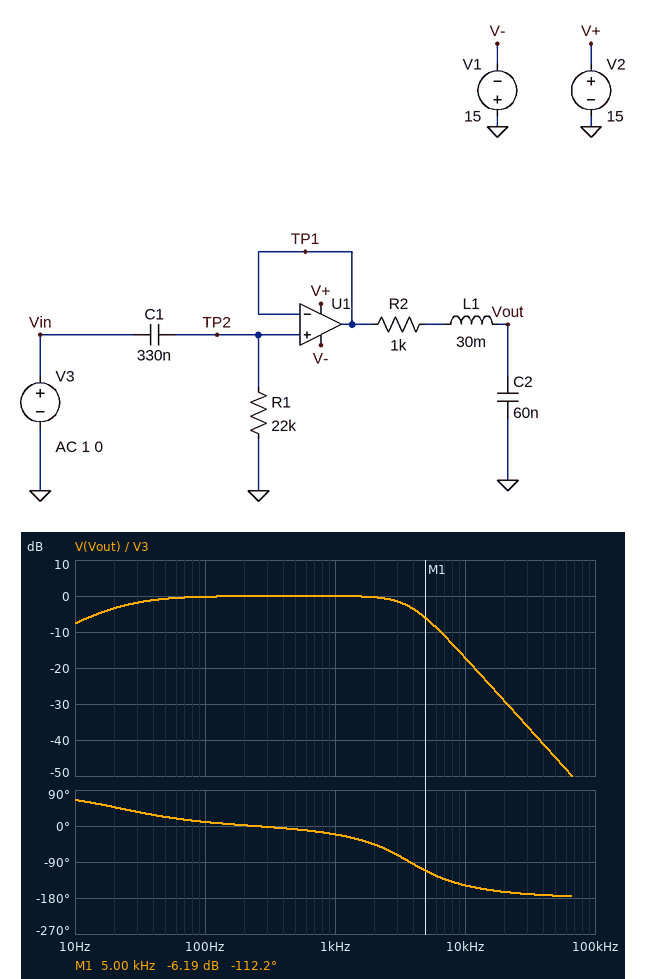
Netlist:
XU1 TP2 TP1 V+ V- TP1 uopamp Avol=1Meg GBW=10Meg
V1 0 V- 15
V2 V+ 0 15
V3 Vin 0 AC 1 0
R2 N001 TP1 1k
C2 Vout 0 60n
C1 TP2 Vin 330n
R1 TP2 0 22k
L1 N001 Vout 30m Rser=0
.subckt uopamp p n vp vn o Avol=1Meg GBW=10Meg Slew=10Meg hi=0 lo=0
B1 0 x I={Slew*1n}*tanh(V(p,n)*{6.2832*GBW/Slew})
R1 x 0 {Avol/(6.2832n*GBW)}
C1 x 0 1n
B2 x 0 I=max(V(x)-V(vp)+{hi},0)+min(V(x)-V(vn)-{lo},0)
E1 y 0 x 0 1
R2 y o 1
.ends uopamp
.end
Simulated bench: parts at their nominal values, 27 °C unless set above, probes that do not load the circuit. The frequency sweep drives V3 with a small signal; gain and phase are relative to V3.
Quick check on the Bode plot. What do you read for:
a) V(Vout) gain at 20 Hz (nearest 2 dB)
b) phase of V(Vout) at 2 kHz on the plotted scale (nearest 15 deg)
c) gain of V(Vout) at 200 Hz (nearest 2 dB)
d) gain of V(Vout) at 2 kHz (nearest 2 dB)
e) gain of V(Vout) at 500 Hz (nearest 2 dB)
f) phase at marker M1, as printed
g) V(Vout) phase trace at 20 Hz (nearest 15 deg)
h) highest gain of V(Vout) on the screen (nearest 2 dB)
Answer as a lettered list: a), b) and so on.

a) -4 dB
b) -45 deg
c) 0 dB
d) 0 dB
e) 0 dB
f) -112.2 deg
g) 45 deg
h) 0 dB
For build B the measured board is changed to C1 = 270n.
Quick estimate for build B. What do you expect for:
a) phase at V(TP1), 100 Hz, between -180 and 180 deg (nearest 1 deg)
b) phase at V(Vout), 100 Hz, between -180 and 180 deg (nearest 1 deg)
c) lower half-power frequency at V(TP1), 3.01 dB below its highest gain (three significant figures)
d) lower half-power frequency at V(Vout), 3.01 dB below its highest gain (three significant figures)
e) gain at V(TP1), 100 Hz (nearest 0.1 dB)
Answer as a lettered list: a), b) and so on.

a) 15 deg
b) 13 deg
c) 26.8 Hz
d) 26.7 Hz
e) -0.3 dB
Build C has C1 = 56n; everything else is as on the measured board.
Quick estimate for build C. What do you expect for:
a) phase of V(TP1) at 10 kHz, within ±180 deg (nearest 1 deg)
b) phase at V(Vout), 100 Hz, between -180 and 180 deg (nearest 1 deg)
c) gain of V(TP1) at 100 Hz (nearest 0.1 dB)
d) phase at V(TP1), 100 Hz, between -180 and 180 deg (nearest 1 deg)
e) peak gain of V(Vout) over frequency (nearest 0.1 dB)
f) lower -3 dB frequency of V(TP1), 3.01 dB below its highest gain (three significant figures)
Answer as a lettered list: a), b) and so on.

a) 1 deg
b) 50 deg
c) -4.3 dB
d) 52 deg
e) -0.1 dB
f) 129 Hz
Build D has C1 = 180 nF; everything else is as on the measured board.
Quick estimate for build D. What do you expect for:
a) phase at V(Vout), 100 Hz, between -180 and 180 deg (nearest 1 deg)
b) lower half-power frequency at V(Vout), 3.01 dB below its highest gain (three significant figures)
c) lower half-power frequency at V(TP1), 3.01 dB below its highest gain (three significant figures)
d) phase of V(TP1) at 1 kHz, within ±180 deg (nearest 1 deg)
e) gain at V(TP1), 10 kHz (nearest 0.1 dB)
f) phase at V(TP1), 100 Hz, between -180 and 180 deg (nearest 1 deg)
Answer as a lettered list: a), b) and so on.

a) 20 deg
b) 40.0 Hz
c) 40.2 Hz
d) 2 deg
e) 0 dB
f) 22 deg
